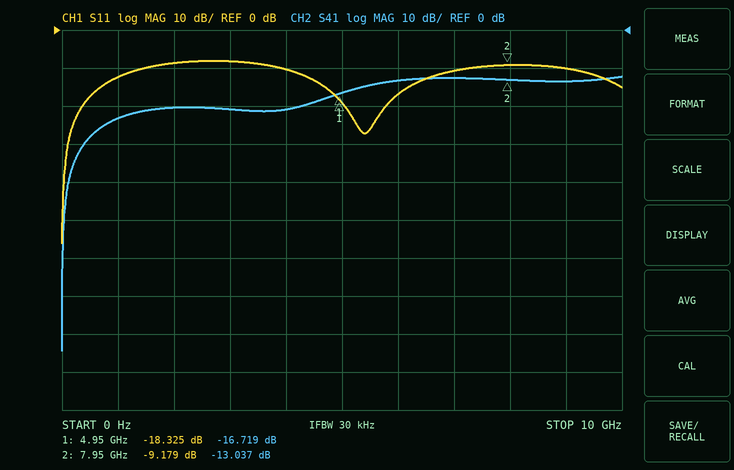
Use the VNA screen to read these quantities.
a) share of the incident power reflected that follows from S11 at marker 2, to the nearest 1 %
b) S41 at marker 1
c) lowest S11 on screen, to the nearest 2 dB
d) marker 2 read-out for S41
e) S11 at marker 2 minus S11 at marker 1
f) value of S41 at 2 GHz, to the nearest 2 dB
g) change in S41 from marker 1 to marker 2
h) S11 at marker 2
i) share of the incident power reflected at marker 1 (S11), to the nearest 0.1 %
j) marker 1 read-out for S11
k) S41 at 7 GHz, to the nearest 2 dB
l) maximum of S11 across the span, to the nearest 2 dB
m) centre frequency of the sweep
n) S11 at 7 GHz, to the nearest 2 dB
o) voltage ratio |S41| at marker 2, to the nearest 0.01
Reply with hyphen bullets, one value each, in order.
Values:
- 12 %
- -16.719 dB
- -56 dB
- -13.037 dB
- 9.146 dB
- -20 dB
- 3.682 dB
- -9.179 dB
- 1.5 %
- -18.325 dB
- -12 dB
- -8 dB
- 5 GHz
- -10 dB
- 0.22
